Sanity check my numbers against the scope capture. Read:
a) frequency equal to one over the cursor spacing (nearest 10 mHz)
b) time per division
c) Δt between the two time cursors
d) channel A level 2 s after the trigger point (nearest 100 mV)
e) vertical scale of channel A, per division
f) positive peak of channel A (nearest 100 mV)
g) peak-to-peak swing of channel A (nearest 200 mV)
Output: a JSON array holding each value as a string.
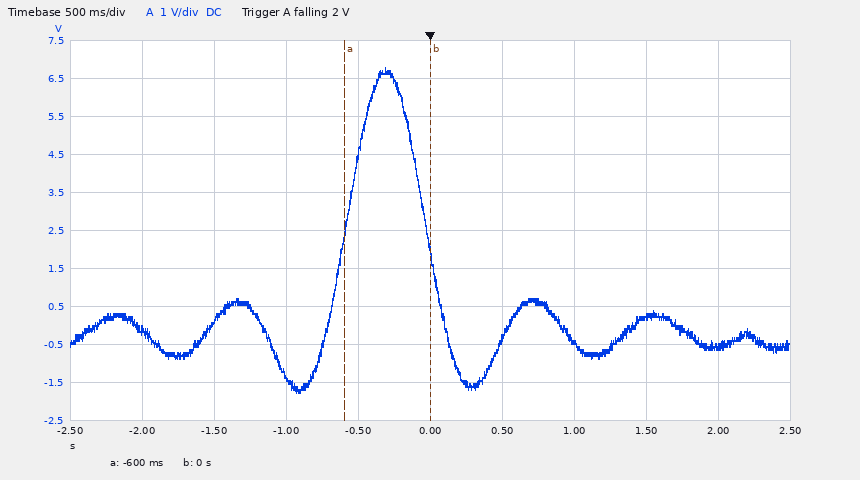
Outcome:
["1.67 Hz", "500 ms", "600 ms", "-600 mV", "1 V", "6.8 V", "8.6 V"]
